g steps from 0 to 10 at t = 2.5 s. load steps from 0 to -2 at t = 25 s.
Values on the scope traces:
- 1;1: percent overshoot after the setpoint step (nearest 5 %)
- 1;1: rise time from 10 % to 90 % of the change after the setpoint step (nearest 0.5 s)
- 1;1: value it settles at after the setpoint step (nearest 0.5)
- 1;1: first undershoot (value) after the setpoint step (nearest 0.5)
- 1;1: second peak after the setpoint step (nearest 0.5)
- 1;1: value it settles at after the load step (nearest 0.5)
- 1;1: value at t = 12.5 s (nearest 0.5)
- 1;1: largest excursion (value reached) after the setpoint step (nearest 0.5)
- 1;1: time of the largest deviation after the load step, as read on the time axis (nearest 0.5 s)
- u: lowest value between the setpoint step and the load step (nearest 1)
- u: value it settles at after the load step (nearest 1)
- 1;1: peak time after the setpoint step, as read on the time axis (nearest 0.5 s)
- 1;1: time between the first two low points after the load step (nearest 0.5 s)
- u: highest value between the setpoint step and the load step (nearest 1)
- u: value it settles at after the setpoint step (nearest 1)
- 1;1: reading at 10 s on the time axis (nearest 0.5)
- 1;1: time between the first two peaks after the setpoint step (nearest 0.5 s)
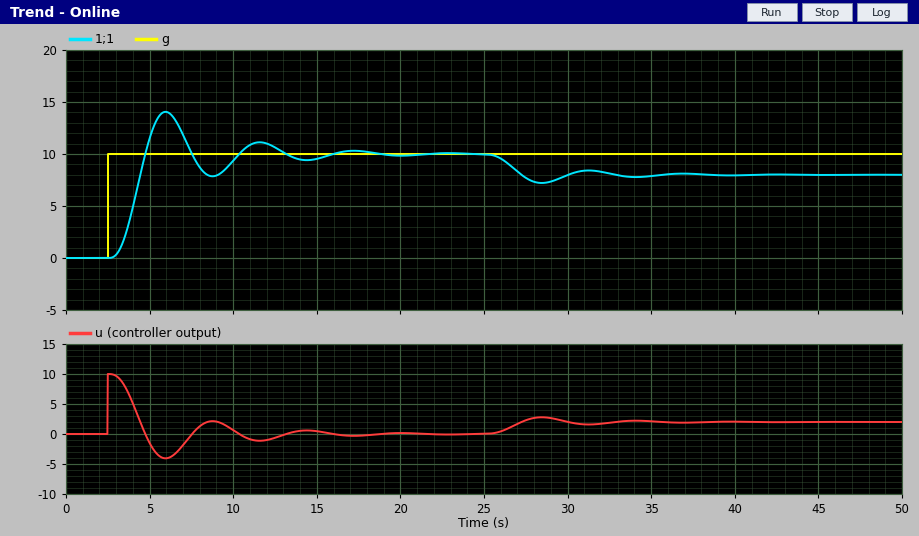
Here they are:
40 %
1.5 s
10.0
8.0
11.0
8.0
10.5
14.0
28.5 s
-4
2
6.0 s
5.5 s
10
0
9.5
5.5 s
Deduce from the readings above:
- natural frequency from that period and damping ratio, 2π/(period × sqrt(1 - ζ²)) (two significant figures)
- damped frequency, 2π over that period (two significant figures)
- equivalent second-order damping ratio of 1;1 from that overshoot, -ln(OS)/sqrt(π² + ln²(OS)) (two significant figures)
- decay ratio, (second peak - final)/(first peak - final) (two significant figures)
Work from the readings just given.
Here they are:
1.2 rad/s
1.1 rad/s
0.28
0.25
